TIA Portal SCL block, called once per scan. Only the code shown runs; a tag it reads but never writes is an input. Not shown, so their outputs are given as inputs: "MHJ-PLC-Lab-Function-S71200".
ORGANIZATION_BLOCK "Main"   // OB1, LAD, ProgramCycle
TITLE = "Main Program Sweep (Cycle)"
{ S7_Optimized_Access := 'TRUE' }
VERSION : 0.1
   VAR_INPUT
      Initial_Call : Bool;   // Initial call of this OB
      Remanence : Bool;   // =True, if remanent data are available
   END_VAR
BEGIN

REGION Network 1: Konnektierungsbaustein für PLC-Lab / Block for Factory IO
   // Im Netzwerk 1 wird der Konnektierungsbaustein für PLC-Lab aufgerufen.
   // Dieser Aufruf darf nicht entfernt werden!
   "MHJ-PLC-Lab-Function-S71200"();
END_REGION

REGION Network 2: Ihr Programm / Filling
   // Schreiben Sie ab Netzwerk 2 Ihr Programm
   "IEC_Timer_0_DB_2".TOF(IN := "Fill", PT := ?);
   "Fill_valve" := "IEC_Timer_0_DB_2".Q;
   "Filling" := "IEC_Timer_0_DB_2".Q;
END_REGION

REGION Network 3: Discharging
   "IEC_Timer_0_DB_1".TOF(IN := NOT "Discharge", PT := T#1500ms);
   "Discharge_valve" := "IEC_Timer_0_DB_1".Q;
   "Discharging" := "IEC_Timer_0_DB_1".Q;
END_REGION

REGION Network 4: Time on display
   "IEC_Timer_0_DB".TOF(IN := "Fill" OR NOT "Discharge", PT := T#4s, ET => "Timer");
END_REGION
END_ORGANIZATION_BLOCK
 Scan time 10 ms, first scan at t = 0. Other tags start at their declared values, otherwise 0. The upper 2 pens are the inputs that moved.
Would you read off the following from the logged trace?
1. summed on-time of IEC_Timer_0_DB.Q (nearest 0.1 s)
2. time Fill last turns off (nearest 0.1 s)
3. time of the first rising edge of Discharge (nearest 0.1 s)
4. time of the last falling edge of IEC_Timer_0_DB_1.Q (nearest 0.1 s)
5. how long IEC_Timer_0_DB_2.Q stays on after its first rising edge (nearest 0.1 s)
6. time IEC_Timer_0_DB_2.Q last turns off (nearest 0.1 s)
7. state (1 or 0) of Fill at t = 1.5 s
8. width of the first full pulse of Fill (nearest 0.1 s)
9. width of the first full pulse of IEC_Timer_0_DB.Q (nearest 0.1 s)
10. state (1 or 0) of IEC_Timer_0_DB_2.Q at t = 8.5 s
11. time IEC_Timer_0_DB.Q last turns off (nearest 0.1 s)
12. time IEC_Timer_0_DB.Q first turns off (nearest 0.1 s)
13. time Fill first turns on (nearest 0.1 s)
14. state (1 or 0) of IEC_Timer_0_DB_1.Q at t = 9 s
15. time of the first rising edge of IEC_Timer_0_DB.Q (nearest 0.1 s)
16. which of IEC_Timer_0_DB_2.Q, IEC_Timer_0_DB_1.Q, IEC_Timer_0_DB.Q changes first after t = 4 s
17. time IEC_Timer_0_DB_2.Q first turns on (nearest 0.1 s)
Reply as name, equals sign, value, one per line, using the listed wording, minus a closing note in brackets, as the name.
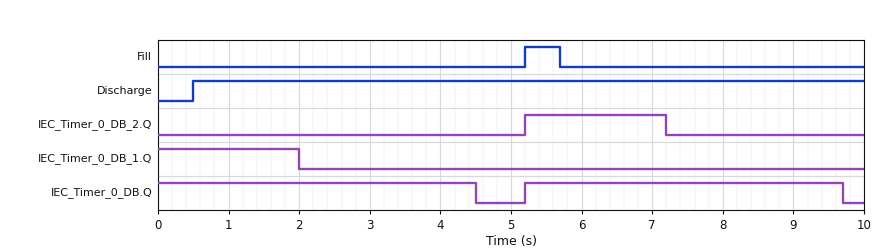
summed on-time of IEC_Timer_0_DB.Q = 9.0 s
time Fill last turns off = 5.7 s
time of the first rising edge of Discharge = 0.5 s
time of the last falling edge of IEC_Timer_0_DB_1.Q = 2.0 s
how long IEC_Timer_0_DB_2.Q stays on after its first rising edge = 2.0 s
time IEC_Timer_0_DB_2.Q last turns off = 7.2 s
state (1 or 0) of Fill at t = 1.5 s = 0
width of the first full pulse of Fill = 0.5 s
width of the first full pulse of IEC_Timer_0_DB.Q = 4.5 s
state (1 or 0) of IEC_Timer_0_DB_2.Q at t = 8.5 s = 0
time IEC_Timer_0_DB.Q last turns off = 9.7 s
time IEC_Timer_0_DB.Q first turns off = 4.5 s
time Fill first turns on = 5.2 s
state (1 or 0) of IEC_Timer_0_DB_1.Q at t = 9 s = 0
time of the first rising edge of IEC_Timer_0_DB.Q = 5.2 s
which of IEC_Timer_0_DB_2.Q, IEC_Timer_0_DB_1.Q, IEC_Timer_0_DB.Q changes first after t = 4 s = IEC_Timer_0_DB.Q
time IEC_Timer_0_DB_2.Q first turns on = 5.2 s
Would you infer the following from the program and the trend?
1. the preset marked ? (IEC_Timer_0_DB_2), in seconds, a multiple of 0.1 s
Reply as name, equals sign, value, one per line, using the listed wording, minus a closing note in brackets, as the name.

the preset marked ? (IEC_Timer_0_DB_2), in seconds, a multiple of 0.1 s = 1.5 s
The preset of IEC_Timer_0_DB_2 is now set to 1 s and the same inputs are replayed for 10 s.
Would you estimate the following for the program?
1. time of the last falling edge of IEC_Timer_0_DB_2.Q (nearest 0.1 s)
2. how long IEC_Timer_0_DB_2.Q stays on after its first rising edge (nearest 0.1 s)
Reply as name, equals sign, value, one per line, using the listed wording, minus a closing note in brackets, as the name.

time of the last falling edge of IEC_Timer_0_DB_2.Q = 6.7 s
how long IEC_Timer_0_DB_2.Q stays on after its first rising edge = 1.5 s
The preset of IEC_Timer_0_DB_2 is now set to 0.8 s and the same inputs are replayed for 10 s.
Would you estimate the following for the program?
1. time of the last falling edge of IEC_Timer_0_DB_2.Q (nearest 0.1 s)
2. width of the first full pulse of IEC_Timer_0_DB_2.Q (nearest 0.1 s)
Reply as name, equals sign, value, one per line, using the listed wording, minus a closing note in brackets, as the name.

time of the last falling edge of IEC_Timer_0_DB_2.Q = 6.5 s
width of the first full pulse of IEC_Timer_0_DB_2.Q = 1.3 s
